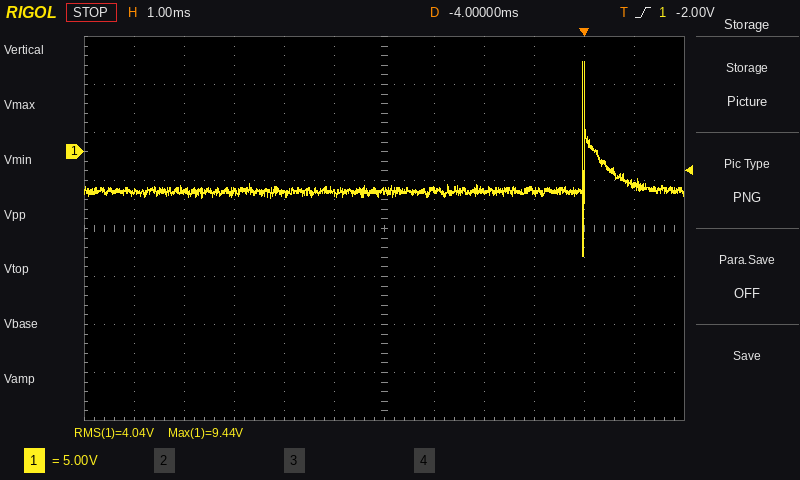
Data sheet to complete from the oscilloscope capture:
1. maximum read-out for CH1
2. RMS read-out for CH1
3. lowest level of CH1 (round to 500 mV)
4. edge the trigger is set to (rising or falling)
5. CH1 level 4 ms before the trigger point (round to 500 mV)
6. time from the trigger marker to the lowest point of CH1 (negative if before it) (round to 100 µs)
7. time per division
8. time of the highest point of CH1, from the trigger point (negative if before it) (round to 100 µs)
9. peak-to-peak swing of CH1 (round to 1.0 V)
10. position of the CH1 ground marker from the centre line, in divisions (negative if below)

9.44 V
4.04 V
-11.0 V
rising
-4.0 V
0.0 ms
1 ms
0.0 ms
20.0 V
+1.6 div
